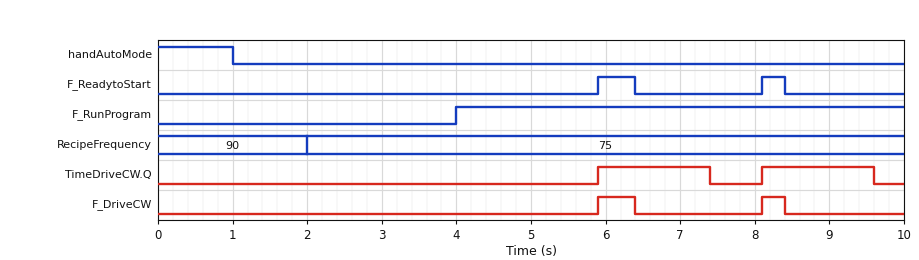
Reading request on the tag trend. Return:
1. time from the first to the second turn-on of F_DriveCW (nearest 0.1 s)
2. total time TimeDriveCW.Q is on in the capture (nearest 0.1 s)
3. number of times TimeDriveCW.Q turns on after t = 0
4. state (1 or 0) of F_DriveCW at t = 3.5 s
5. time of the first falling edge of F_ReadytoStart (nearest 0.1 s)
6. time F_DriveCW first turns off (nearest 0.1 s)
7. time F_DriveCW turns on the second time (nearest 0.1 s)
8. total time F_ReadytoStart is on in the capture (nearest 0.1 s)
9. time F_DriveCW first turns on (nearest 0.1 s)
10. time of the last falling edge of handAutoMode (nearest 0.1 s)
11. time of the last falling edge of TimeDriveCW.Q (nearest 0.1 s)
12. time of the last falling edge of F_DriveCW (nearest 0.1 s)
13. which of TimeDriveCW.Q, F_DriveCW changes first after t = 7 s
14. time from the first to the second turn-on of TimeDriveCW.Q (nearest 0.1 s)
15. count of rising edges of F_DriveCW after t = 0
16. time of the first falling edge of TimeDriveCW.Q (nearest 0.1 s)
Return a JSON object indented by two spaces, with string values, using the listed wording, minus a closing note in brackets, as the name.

{
  "time from the first to the second turn-on of F_DriveCW": "2.2 s",
  "total time TimeDriveCW.Q is on in the capture": "3.0 s",
  "number of times TimeDriveCW.Q turns on after t = 0": "2",
  "state (1 or 0) of F_DriveCW at t = 3.5 s": "0",
  "time of the first falling edge of F_ReadytoStart": "6.4 s",
  "time F_DriveCW first turns off": "6.4 s",
  "time F_DriveCW turns on the second time": "8.1 s",
  "total time F_ReadytoStart is on in the capture": "0.8 s",
  "time F_DriveCW first turns on": "5.9 s",
  "time of the last falling edge of handAutoMode": "1.0 s",
  "time of the last falling edge of TimeDriveCW.Q": "9.6 s",
  "time of the last falling edge of F_DriveCW": "8.4 s",
  "which of TimeDriveCW.Q, F_DriveCW changes first after t = 7 s": "TimeDriveCW.Q",
  "time from the first to the second turn-on of TimeDriveCW.Q": "2.2 s",
  "count of rising edges of F_DriveCW after t = 0": "2",
  "time of the first falling edge of TimeDriveCW.Q": "7.4 s"
}
